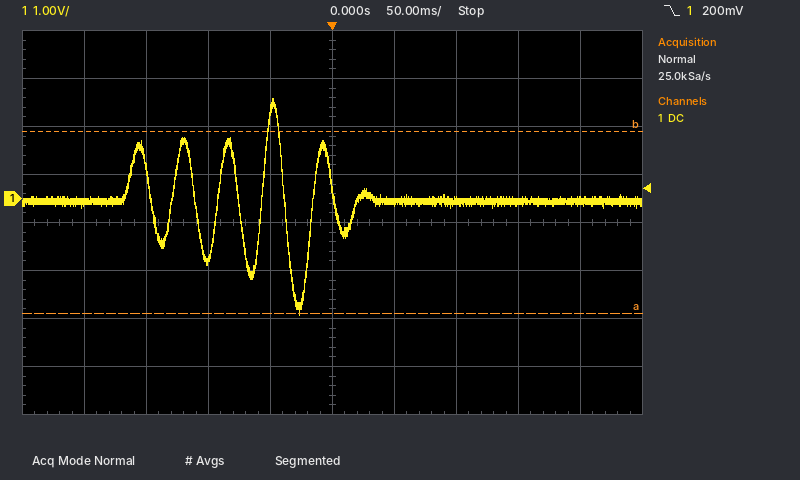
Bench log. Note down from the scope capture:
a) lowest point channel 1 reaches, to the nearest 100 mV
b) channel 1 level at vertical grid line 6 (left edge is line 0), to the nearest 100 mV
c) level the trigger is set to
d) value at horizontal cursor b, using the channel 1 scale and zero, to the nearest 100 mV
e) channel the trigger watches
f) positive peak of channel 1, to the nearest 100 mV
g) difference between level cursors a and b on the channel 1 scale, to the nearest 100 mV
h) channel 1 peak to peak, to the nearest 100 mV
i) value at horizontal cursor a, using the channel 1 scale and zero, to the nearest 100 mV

-2.4 V
-100 mV
200 mV
1.4 V
channel 1
2.1 V
3.8 V
4.5 V
-2.4 V
